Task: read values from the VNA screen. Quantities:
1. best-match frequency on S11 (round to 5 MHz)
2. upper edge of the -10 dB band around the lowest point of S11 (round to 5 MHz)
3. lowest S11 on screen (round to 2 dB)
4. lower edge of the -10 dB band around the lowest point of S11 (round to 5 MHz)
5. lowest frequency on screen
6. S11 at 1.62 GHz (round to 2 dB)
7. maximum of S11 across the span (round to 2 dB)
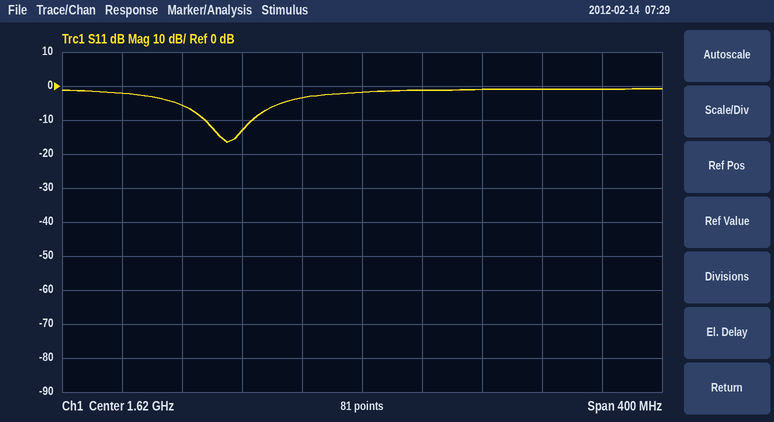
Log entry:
1.530 GHz
1.545 GHz
-16 dB
1.515 GHz
1.42 GHz
-2 dB
0 dB
